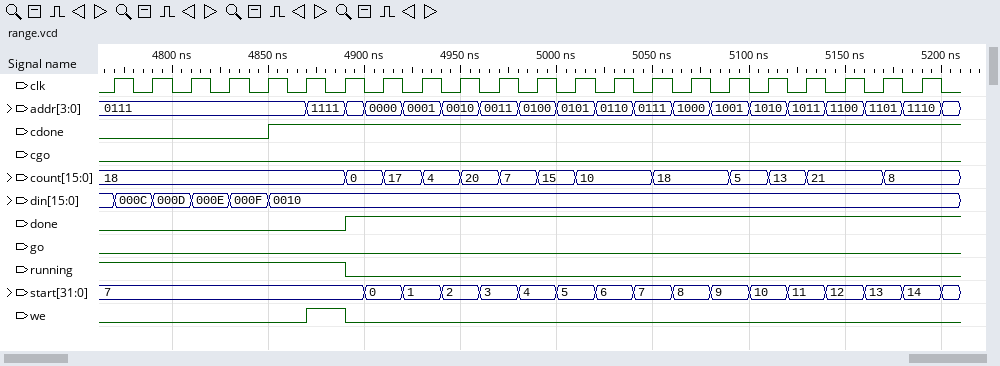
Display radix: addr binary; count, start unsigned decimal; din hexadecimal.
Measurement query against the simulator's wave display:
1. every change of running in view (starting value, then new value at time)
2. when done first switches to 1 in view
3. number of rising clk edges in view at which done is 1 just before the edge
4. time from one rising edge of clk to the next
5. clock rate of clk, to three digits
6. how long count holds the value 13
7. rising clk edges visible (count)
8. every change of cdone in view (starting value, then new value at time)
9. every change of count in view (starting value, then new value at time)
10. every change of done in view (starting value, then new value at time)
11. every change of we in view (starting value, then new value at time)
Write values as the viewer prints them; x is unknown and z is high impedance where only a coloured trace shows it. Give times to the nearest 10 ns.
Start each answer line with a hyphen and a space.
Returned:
- 1, 0 at 4890 ns
- 4890 ns
- 15
- 20 ns
- 50.0 MHz
- 20 ns
- 22
- 0, 1 at 4850 ns
- 18, 0 at 4890 ns, 17 at 4910 ns, 4 at 4930 ns, 20 at 4950 ns, 7 at 4970 ns, 15 at 4990 ns, 10 at 5010 ns, 18 at 5050 ns, 5 at 5090 ns, 13 at 5110 ns, 21 at 5130 ns, 8 at 5170 ns
- 0, 1 at 4890 ns
- 0, 1 at 4870 ns, 0 at 4890 ns
